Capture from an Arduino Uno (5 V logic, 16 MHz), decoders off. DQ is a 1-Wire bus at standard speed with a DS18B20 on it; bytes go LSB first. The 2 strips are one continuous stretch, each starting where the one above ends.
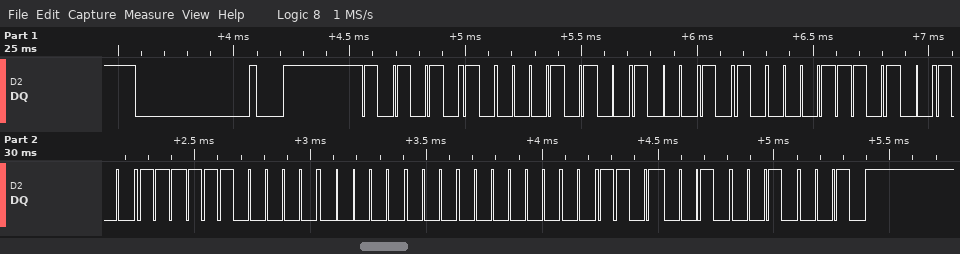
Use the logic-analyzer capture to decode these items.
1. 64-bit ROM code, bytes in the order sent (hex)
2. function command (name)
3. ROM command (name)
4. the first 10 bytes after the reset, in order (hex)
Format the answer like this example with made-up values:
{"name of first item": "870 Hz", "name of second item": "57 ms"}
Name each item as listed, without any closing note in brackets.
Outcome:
{"64-bit ROM code, bytes in the order sent": "28 51 B8 E4 07 00 00 4B", "function command": "Convert T", "ROM command": "Match ROM", "the first 10 bytes after the reset, in order": "55 28 51 B8 E4 07 00 00 4B 44"}
